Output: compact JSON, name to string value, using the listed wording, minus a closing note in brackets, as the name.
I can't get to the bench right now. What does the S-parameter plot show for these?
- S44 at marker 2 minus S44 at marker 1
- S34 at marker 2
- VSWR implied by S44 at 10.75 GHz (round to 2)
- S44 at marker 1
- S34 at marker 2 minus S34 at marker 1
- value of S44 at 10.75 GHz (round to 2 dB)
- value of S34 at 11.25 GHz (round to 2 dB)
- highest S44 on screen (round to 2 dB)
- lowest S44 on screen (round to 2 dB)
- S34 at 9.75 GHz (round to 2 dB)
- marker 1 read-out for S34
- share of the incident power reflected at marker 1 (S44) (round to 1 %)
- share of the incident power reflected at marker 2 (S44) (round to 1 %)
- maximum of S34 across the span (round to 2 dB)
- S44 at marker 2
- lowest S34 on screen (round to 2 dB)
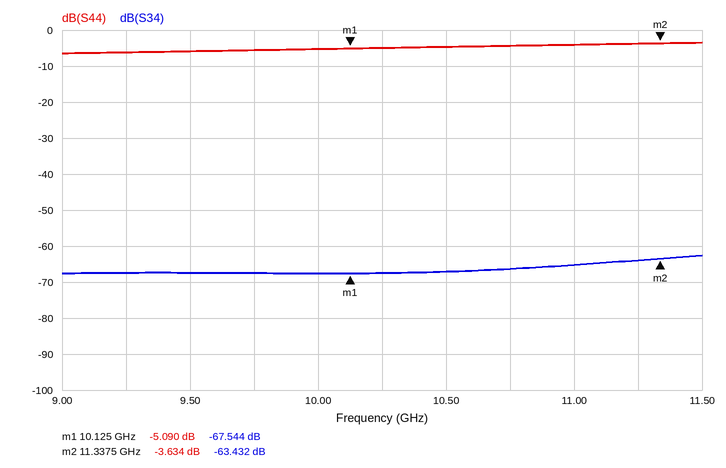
{"S44 at marker 2 minus S44 at marker 1": "1.456 dB", "S34 at marker 2": "-63.432 dB", "VSWR implied by S44 at 10.75 GHz": "4", "S44 at marker 1": "-5.090 dB", "S34 at marker 2 minus S34 at marker 1": "4.112 dB", "value of S44 at 10.75 GHz": "-4 dB", "value of S34 at 11.25 GHz": "-64 dB", "highest S44 on screen": "-4 dB", "lowest S44 on screen": "-6 dB", "S34 at 9.75 GHz": "-68 dB", "marker 1 read-out for S34": "-67.544 dB", "share of the incident power reflected at marker 1 (S44)": "31 %", "share of the incident power reflected at marker 2 (S44)": "43 %", "maximum of S34 across the span": "-62 dB", "S44 at marker 2": "-3.634 dB", "lowest S34 on screen": "-68 dB"}
